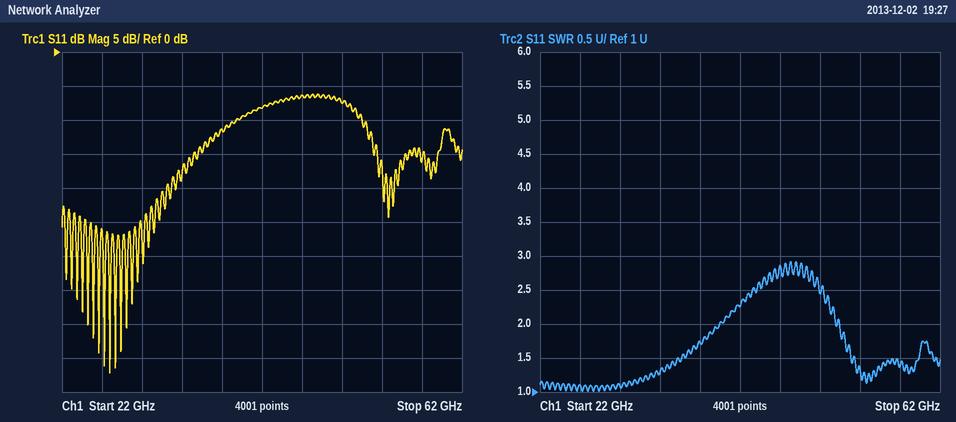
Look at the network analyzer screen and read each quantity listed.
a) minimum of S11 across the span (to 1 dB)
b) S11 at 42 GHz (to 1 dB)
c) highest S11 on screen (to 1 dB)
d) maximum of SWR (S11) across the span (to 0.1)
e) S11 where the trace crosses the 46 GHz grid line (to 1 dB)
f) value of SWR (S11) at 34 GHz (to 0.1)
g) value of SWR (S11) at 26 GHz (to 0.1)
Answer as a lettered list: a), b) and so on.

a) -47 dB
b) -8 dB
c) -6 dB
d) 2.9
e) -6 dB
f) 1.3
g) 1.1
